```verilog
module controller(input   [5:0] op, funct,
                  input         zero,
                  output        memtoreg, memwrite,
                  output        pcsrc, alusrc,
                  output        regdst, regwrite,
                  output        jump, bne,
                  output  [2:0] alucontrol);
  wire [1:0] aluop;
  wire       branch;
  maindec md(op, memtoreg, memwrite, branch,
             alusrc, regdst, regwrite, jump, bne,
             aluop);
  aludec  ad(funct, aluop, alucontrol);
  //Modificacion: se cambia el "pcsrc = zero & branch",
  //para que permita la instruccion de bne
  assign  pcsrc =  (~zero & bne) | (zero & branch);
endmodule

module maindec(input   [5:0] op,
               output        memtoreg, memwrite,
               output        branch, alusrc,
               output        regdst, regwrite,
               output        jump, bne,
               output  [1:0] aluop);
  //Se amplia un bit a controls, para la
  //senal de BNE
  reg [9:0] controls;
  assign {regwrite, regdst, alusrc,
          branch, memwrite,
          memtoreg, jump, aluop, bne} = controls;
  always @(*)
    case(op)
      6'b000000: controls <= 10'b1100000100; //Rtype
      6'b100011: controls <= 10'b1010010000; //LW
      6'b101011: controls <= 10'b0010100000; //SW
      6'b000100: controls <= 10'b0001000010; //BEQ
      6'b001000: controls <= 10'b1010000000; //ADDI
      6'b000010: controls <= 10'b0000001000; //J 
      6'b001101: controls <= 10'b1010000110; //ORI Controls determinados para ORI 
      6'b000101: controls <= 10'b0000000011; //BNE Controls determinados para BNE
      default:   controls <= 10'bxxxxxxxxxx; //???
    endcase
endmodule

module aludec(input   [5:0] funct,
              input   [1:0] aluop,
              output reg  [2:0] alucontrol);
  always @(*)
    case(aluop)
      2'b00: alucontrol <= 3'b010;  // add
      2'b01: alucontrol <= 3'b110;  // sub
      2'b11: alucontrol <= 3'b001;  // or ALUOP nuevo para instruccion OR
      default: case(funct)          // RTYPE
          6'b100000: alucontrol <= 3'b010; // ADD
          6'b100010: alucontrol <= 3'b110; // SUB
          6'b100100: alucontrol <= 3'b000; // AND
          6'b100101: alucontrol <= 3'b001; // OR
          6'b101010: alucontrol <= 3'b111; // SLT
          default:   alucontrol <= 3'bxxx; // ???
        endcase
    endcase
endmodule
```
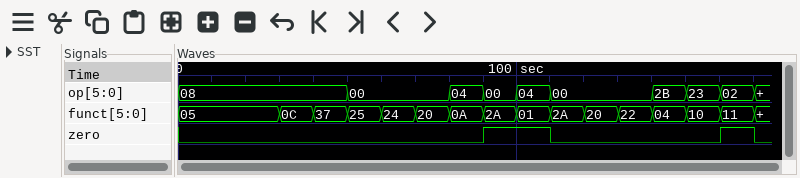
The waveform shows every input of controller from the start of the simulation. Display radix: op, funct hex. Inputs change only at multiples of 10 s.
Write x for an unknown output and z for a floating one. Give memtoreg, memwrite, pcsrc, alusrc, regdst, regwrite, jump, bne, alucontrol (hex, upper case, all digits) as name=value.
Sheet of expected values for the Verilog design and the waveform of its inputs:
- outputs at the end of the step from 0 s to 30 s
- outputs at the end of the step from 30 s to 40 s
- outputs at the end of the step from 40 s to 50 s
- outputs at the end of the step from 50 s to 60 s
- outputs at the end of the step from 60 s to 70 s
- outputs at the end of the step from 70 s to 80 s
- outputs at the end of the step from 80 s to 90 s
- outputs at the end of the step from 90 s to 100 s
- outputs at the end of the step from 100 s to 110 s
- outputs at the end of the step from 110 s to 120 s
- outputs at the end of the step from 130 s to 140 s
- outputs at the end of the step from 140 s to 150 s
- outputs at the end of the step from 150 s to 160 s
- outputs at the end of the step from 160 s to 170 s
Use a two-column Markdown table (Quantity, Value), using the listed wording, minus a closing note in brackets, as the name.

| Quantity | Value |
|---|---|
| outputs at the end of the step from 0 s to 30 s | memtoreg=0, memwrite=0, pcsrc=0, alusrc=1, regdst=0, regwrite=1, jump=0, bne=0, alucontrol=2 |
| outputs at the end of the step from 30 s to 40 s | memtoreg=0, memwrite=0, pcsrc=0, alusrc=1, regdst=0, regwrite=1, jump=0, bne=0, alucontrol=2 |
| outputs at the end of the step from 40 s to 50 s | memtoreg=0, memwrite=0, pcsrc=0, alusrc=1, regdst=0, regwrite=1, jump=0, bne=0, alucontrol=2 |
| outputs at the end of the step from 50 s to 60 s | memtoreg=0, memwrite=0, pcsrc=0, alusrc=0, regdst=1, regwrite=1, jump=0, bne=0, alucontrol=1 |
| outputs at the end of the step from 60 s to 70 s | memtoreg=0, memwrite=0, pcsrc=0, alusrc=0, regdst=1, regwrite=1, jump=0, bne=0, alucontrol=0 |
| outputs at the end of the step from 70 s to 80 s | memtoreg=0, memwrite=0, pcsrc=0, alusrc=0, regdst=1, regwrite=1, jump=0, bne=0, alucontrol=2 |
| outputs at the end of the step from 80 s to 90 s | memtoreg=0, memwrite=0, pcsrc=0, alusrc=0, regdst=0, regwrite=0, jump=0, bne=0, alucontrol=6 |
| outputs at the end of the step from 90 s to 100 s | memtoreg=0, memwrite=0, pcsrc=0, alusrc=0, regdst=1, regwrite=1, jump=0, bne=0, alucontrol=7 |
| outputs at the end of the step from 100 s to 110 s | memtoreg=0, memwrite=0, pcsrc=1, alusrc=0, regdst=0, regwrite=0, jump=0, bne=0, alucontrol=6 |
| outputs at the end of the step from 110 s to 120 s | memtoreg=0, memwrite=0, pcsrc=0, alusrc=0, regdst=1, regwrite=1, jump=0, bne=0, alucontrol=7 |
| outputs at the end of the step from 130 s to 140 s | memtoreg=0, memwrite=0, pcsrc=0, alusrc=0, regdst=1, regwrite=1, jump=0, bne=0, alucontrol=6 |
| outputs at the end of the step from 140 s to 150 s | memtoreg=0, memwrite=1, pcsrc=0, alusrc=1, regdst=0, regwrite=0, jump=0, bne=0, alucontrol=2 |
| outputs at the end of the step from 150 s to 160 s | memtoreg=1, memwrite=0, pcsrc=0, alusrc=1, regdst=0, regwrite=1, jump=0, bne=0, alucontrol=2 |
| outputs at the end of the step from 160 s to 170 s | memtoreg=0, memwrite=0, pcsrc=0, alusrc=0, regdst=0, regwrite=0, jump=1, bne=0, alucontrol=2 |
